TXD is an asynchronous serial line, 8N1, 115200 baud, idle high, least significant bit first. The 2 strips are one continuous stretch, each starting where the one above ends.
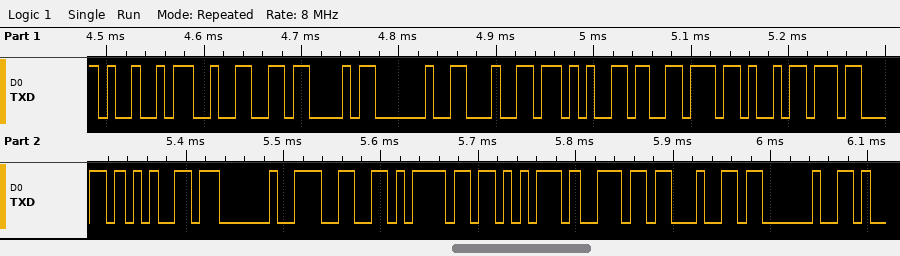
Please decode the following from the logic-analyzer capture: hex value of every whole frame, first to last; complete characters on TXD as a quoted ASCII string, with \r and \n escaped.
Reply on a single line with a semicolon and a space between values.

0x49 0x32 0x43 0x20 0x64 0x65 0x76 0x69 0x63 0x65 0x20 0x66 0x6F 0x75 0x6E 0x64 0x20; "I2C device found "
